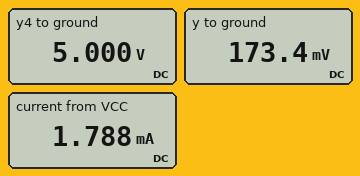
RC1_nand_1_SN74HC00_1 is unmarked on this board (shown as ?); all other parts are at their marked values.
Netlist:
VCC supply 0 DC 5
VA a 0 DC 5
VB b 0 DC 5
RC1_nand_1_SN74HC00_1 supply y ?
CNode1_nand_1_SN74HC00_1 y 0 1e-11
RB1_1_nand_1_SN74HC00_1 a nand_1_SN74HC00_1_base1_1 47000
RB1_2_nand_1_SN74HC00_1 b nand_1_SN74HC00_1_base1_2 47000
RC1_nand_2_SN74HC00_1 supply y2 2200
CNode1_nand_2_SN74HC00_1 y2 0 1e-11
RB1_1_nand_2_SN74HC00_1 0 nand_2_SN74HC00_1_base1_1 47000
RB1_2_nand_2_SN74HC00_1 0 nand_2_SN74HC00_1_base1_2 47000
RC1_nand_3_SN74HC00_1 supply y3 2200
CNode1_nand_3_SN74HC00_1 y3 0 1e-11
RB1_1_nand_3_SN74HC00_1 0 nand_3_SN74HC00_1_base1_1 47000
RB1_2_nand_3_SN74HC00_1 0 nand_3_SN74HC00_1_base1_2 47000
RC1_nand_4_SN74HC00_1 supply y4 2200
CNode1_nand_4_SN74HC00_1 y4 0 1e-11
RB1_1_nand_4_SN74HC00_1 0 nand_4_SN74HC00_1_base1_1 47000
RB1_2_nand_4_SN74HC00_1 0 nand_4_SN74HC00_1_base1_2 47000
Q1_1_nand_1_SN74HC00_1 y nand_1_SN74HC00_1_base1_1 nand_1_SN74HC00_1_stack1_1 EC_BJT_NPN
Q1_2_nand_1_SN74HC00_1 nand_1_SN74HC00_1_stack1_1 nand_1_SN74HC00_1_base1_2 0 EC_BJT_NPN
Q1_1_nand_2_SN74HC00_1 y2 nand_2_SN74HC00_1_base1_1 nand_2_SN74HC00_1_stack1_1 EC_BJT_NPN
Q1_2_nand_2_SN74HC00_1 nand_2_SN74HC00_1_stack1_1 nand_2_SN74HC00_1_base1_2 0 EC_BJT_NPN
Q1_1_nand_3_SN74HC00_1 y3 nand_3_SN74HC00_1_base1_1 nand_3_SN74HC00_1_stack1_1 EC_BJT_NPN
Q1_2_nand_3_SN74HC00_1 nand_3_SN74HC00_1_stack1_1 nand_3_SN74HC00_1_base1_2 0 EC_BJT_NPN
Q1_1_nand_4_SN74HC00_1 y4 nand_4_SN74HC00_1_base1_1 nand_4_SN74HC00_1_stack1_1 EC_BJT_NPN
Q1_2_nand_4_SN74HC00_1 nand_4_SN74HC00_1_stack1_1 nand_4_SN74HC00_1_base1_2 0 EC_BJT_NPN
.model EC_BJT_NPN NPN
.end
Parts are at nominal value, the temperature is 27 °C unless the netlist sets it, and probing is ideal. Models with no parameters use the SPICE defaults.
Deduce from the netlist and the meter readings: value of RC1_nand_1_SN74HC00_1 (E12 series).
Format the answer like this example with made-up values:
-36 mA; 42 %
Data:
2.7 kΩ
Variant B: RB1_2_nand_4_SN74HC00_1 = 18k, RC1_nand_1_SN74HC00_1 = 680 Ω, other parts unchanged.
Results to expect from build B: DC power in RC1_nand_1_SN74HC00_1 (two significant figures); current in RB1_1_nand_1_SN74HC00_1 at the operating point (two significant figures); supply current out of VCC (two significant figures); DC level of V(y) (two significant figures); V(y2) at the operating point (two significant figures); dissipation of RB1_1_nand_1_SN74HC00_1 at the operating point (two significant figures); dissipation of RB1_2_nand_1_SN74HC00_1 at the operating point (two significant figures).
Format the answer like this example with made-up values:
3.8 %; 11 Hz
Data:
32 mW; 86 µA; 6.9 mA; 310 mV; 5.0 V; 340 µW; 370 µW
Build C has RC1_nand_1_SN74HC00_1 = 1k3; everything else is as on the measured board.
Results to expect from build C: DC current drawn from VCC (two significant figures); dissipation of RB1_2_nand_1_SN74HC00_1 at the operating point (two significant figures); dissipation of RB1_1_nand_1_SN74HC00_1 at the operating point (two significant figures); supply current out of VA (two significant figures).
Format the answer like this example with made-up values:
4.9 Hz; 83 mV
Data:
3.7 mA; 370 µW; 350 µW; 87 µA
